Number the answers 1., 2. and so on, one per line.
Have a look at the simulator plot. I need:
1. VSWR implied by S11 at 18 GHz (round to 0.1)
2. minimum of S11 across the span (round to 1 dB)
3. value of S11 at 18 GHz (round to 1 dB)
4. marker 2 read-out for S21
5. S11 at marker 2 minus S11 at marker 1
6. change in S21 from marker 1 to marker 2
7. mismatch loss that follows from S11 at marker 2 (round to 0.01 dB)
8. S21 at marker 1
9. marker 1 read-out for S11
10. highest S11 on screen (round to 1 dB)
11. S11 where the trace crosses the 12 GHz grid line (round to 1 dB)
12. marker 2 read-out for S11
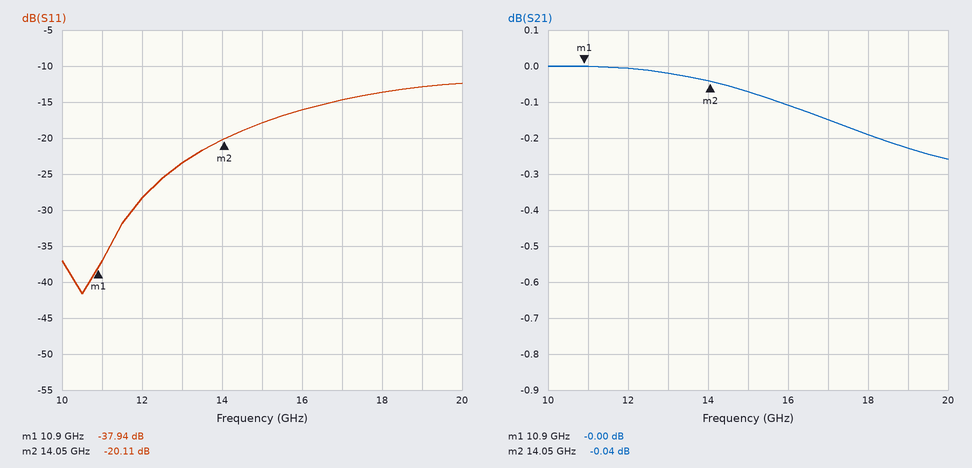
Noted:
1. 1.5
2. -42 dB
3. -14 dB
4. -0.04 dB
5. 17.83 dB
6. -0.04 dB
7. 0.04 dB
8. -0.00 dB
9. -37.94 dB
10. -12 dB
11. -28 dB
12. -20.11 dB
